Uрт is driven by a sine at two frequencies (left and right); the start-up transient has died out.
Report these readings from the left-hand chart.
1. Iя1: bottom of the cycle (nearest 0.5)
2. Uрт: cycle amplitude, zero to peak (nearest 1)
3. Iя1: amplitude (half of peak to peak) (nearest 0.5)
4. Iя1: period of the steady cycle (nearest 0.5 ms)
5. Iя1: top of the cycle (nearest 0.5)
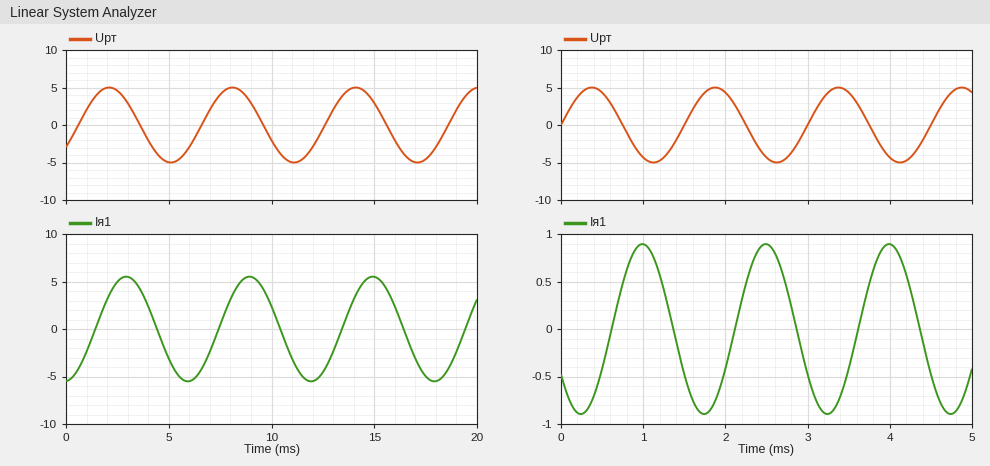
-5.5
5
5.5
6.0 ms
5.5
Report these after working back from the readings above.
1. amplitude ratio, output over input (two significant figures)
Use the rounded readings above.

1.1
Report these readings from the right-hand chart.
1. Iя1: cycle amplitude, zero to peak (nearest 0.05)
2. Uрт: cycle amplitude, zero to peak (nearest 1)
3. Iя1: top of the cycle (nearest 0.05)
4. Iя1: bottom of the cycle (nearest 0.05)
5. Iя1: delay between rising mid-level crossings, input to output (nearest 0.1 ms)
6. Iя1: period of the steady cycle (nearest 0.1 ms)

0.90
5
0.90
-0.90
0.6 ms
1.5 ms
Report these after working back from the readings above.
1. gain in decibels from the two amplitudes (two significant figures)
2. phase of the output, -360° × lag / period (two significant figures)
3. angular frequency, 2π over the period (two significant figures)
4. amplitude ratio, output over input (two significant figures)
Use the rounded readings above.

-15 dB
-140°
4.2 rad/ms
0.18
